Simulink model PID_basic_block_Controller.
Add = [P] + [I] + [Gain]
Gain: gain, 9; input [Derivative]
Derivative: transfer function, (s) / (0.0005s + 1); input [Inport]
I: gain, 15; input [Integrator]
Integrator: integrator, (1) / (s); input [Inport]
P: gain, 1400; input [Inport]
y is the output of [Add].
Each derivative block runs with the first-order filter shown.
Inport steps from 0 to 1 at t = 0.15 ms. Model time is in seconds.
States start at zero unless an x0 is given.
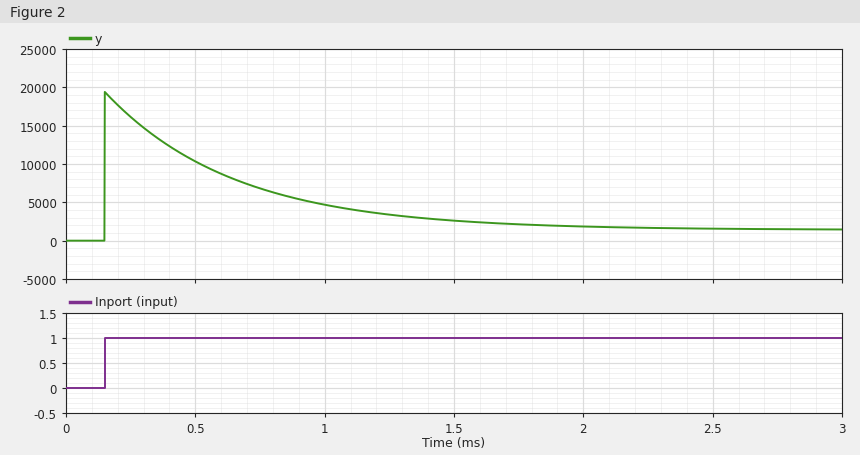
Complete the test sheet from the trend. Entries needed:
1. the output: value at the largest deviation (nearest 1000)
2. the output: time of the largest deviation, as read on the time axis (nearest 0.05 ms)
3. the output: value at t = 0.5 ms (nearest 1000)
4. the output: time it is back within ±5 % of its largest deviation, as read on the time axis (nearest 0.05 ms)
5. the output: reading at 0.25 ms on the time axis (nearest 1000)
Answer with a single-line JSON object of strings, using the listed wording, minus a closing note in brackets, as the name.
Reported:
{"the output: value at the largest deviation": "19000", "the output: time of the largest deviation, as read on the time axis": "0.15 ms", "the output: value at t = 0.5 ms": "10000", "the output: time it is back within ±5 % of its largest deviation, as read on the time axis": "1.60 ms", "the output: reading at 0.25 ms on the time axis": "16000"}
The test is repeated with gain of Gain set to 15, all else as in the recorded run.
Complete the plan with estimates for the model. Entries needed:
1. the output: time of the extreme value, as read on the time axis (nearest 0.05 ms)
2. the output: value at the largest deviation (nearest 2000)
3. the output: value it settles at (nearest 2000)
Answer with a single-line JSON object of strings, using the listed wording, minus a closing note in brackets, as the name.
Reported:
{"the output: time of the extreme value, as read on the time axis": "0.15 ms", "the output: value at the largest deviation": "32000", "the output: value it settles at": "2000"}
